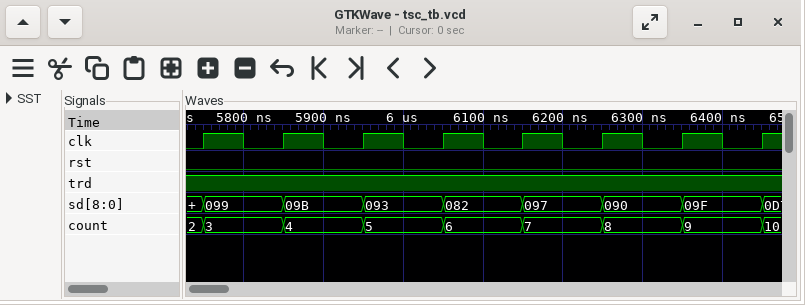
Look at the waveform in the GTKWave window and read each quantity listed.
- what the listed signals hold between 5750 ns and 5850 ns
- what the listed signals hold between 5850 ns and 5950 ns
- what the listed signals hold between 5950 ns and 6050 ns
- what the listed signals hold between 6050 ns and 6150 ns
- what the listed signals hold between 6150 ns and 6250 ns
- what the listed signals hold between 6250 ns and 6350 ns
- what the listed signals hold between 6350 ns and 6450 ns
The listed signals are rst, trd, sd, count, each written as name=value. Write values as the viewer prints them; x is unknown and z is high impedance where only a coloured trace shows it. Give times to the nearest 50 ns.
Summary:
rst=0, trd=1, sd=099, count=3
rst=0, trd=1, sd=09B, count=4
rst=0, trd=1, sd=093, count=5
rst=0, trd=1, sd=082, count=6
rst=0, trd=1, sd=097, count=7
rst=0, trd=1, sd=090, count=8
rst=0, trd=1, sd=09F, count=9
